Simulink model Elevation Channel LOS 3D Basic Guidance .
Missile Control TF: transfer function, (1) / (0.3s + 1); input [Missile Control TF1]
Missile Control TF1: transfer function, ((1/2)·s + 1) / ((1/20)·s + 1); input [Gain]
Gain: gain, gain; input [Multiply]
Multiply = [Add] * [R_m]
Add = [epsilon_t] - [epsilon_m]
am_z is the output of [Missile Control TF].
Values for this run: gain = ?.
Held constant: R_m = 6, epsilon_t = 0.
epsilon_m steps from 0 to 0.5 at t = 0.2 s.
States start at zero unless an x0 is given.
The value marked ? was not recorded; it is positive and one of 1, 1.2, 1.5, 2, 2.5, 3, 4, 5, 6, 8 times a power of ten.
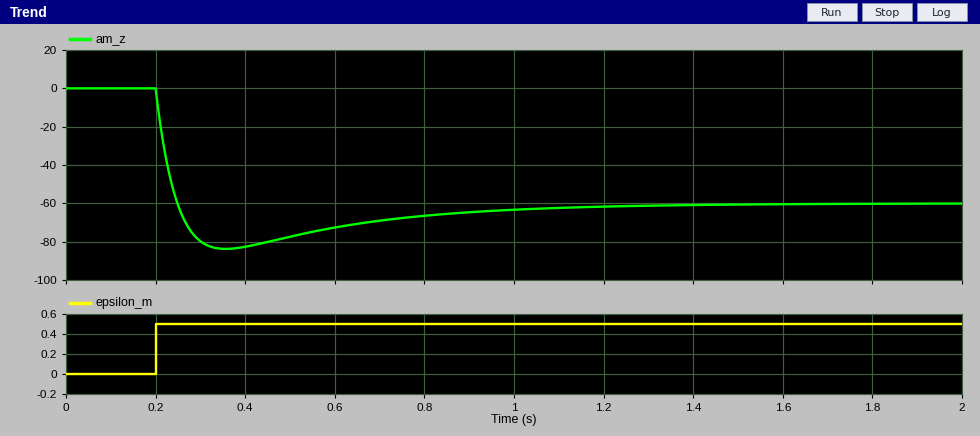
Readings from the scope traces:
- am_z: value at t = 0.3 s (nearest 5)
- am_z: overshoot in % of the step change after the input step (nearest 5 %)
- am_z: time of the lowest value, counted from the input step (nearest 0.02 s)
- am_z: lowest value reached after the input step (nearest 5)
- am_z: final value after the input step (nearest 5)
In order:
-80
40 %
0.16 s
-85
-60
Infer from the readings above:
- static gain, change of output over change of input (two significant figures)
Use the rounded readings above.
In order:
-120
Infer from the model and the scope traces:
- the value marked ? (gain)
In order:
20
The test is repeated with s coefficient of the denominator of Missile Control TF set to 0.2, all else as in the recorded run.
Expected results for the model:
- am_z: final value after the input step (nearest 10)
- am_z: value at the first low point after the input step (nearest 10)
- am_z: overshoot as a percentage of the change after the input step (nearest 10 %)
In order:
-60
-110
80 %
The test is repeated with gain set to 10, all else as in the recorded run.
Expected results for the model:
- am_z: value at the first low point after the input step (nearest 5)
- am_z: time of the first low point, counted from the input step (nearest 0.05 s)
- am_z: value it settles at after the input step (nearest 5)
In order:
-40
0.15 s
-30
